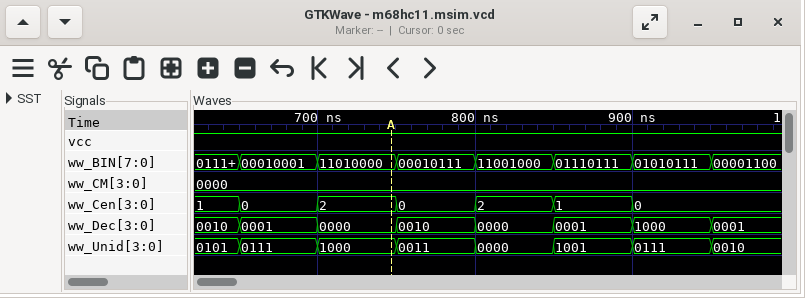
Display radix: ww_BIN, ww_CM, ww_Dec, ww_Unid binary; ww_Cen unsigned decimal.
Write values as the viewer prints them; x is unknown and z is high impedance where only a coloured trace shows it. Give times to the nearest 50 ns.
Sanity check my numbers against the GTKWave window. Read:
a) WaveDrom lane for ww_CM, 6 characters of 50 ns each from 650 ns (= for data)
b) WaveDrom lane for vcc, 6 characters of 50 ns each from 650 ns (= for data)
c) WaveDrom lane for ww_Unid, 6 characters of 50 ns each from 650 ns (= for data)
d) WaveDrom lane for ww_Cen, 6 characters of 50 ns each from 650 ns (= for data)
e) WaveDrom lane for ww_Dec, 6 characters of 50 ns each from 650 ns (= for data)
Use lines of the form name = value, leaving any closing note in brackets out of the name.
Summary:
WaveDrom lane for ww_CM, 6 characters of 50 ns each from 650 ns = {name: 'ww_CM', wave: '=.....', data: '0000'}
WaveDrom lane for vcc, 6 characters of 50 ns each from 650 ns = {name: 'vcc', wave: '1.....'}
WaveDrom lane for ww_Unid, 6 characters of 50 ns each from 650 ns = {name: 'ww_Unid', wave: '======', data: '0111 1000 0011 0000 1001 0111'}
WaveDrom lane for ww_Cen, 6 characters of 50 ns each from 650 ns = {name: 'ww_Cen', wave: '======', data: '0 2 0 2 1 0'}
WaveDrom lane for ww_Dec, 6 characters of 50 ns each from 650 ns = {name: 'ww_Dec', wave: '======', data: '0001 0000 0010 0000 0001 1000'}
